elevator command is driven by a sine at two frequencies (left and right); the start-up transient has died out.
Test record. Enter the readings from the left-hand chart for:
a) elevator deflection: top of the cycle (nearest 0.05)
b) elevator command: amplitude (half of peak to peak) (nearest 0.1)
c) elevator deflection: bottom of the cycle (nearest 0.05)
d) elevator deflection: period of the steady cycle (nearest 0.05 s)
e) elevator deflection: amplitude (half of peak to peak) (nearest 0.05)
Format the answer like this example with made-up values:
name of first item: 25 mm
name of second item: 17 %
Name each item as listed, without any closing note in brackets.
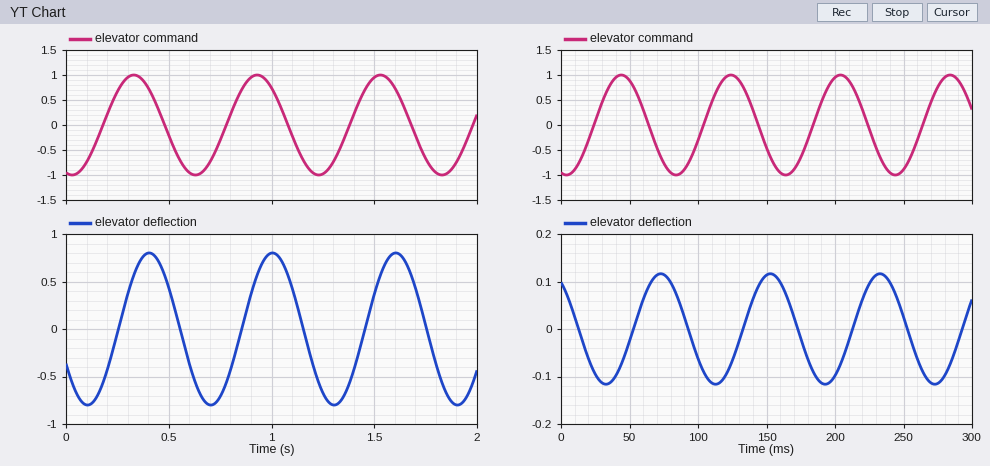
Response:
elevator deflection: top of the cycle: 0.80
elevator command: amplitude (half of peak to peak): 1.0
elevator deflection: bottom of the cycle: -0.80
elevator deflection: period of the steady cycle: 0.60 s
elevator deflection: amplitude (half of peak to peak): 0.80
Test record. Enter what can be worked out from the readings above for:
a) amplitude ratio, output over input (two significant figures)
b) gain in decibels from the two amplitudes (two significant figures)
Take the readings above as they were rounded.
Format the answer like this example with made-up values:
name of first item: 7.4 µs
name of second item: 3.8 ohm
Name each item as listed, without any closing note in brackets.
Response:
amplitude ratio, output over input: 0.80
gain in decibels from the two amplitudes: -1.9 dB
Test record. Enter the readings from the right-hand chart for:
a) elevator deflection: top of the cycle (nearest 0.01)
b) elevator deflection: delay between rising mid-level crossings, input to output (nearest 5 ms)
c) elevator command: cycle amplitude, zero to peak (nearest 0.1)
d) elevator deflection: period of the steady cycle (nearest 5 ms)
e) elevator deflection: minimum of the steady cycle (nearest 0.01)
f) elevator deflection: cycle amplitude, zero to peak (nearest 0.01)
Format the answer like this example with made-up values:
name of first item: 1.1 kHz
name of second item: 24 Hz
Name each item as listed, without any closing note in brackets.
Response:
elevator deflection: top of the cycle: 0.12
elevator deflection: delay between rising mid-level crossings, input to output: 30 ms
elevator command: cycle amplitude, zero to peak: 1.0
elevator deflection: period of the steady cycle: 80 ms
elevator deflection: minimum of the steady cycle: -0.12
elevator deflection: cycle amplitude, zero to peak: 0.12
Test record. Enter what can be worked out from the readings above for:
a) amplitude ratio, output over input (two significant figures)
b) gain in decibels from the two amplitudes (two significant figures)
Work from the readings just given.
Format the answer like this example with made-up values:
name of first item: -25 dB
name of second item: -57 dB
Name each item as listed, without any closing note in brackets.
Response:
amplitude ratio, output over input: 0.12
gain in decibels from the two amplitudes: -18 dB
